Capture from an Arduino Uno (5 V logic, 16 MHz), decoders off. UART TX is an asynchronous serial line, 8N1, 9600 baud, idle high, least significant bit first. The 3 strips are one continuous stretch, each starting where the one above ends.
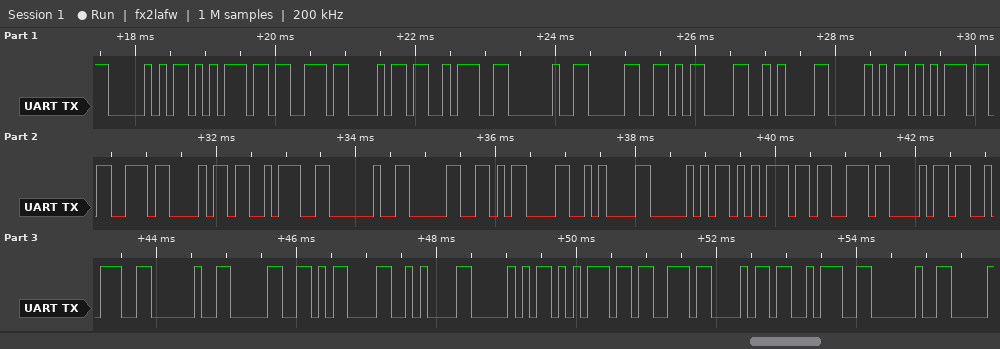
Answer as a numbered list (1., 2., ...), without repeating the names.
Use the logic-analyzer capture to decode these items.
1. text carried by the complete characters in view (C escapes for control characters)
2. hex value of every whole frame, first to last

1. "Push: 0\r\nPush: 0\r\nPush: 0\r\nPush: "
2. 0x50 0x75 0x73 0x68 0x3A 0x20 0x30 0x0D 0x0A 0x50 0x75 0x73 0x68 0x3A 0x20 0x30 0x0D 0x0A 0x50 0x75 0x73 0x68 0x3A 0x20 0x30 0x0D 0x0A 0x50 0x75 0x73 0x68 0x3A 0x20
